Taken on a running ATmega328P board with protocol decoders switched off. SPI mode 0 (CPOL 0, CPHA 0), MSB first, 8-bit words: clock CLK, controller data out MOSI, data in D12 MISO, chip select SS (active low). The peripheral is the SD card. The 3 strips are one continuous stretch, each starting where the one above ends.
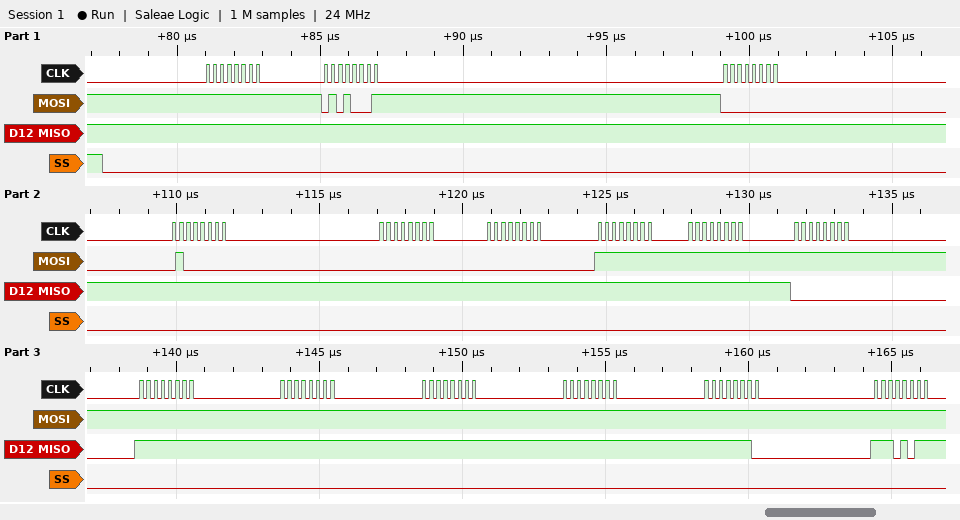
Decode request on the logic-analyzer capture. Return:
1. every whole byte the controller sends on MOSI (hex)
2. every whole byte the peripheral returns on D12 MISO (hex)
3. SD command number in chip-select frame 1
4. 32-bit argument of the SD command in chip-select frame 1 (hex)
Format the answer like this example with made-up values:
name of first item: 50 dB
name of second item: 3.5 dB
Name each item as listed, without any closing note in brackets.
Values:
every whole byte the controller sends on MOSI: FF 51 00 40 00 00 FF FF FF FF FF FF FF FF FF
every whole byte the peripheral returns on D12 MISO: FF FF FF FF FF FF FF FF 00 FF FF FF FF FE EB
SD command number in chip-select frame 1: CMD17
32-bit argument of the SD command in chip-select frame 1: 0x00400000
